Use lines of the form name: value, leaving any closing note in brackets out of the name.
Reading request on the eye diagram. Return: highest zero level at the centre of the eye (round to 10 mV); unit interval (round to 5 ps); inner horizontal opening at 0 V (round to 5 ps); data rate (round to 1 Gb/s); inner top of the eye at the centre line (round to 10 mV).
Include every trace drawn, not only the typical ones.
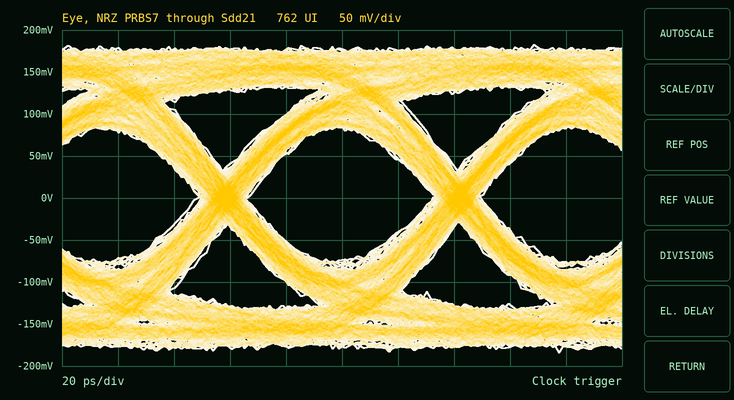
highest zero level at the centre of the eye: -70 mV
unit interval: 85 ps
inner horizontal opening at 0 V: 65 ps
data rate: 12 Gb/s
inner top of the eye at the centre line: 80 mV
